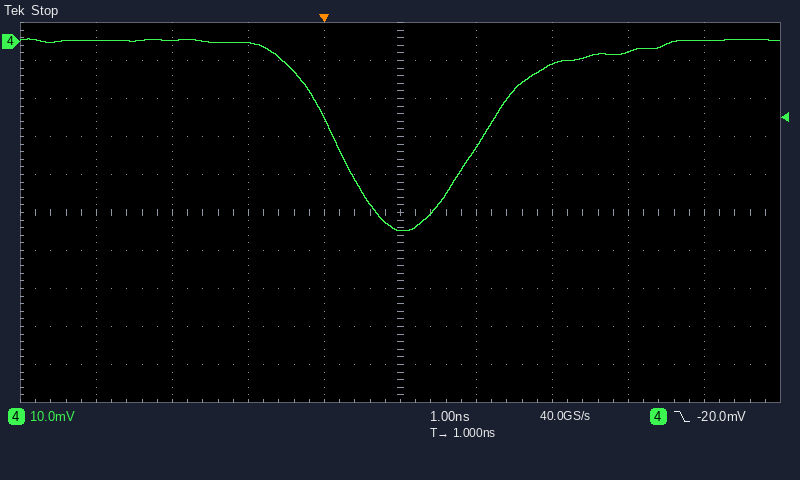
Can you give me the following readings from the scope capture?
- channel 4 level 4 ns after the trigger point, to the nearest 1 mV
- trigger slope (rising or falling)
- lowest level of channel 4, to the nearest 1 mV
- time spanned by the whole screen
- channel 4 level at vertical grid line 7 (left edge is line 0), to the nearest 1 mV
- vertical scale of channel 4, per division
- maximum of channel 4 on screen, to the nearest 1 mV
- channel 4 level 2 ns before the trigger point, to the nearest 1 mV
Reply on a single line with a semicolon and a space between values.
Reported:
-3 mV; falling; -50 mV; 10 ns; -6 mV; 10 mV; 1 mV; 0 mV
